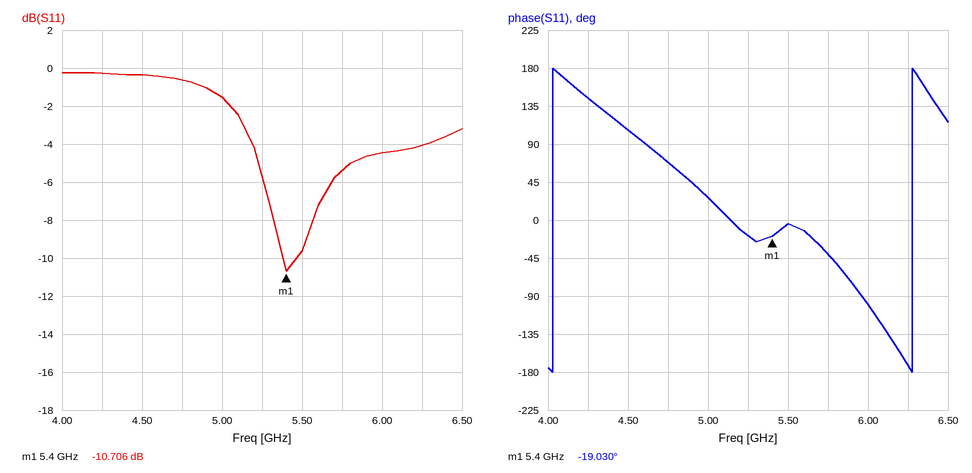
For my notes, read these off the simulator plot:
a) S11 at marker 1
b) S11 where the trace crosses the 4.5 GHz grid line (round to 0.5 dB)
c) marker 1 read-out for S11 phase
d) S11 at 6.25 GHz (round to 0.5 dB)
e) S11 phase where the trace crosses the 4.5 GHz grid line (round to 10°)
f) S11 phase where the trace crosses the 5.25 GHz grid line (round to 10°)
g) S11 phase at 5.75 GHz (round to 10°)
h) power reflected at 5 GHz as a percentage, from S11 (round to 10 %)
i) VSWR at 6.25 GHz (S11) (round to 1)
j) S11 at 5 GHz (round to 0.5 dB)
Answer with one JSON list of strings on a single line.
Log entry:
["-10.706 dB", "-0.5 dB", "-19.030°", "-4.0 dB", "110°", "-20°", "-40°", "70 %", "4", "-1.5 dB"]
